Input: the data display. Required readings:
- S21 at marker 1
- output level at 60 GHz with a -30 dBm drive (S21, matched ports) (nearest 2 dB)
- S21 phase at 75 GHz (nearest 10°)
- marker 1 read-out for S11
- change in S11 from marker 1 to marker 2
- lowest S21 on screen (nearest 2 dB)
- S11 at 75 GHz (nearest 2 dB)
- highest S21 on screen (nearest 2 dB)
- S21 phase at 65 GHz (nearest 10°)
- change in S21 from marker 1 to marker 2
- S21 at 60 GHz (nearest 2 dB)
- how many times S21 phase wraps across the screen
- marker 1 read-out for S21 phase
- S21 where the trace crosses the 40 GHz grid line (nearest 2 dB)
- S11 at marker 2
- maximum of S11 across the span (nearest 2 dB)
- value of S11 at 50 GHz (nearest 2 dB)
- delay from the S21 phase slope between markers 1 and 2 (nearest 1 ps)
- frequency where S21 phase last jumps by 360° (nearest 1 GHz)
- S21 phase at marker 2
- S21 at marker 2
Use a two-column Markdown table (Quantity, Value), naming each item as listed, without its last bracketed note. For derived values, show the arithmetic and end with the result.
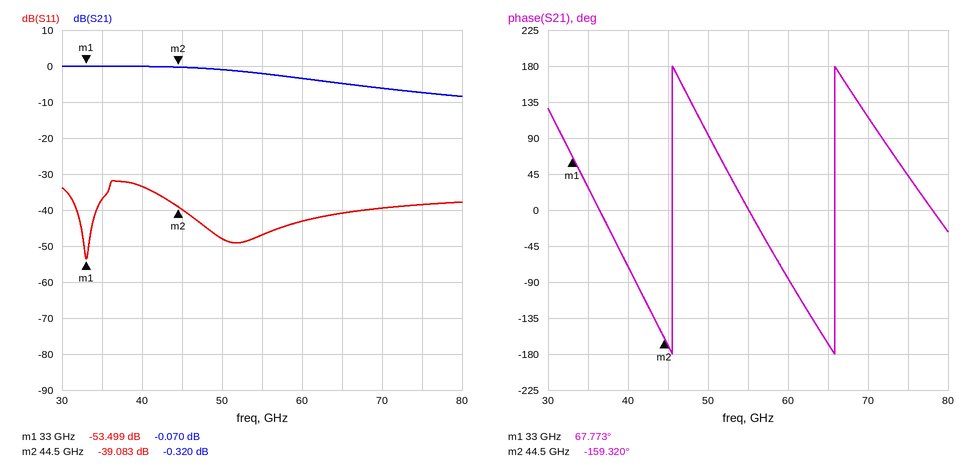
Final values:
| Quantity | Value |
|---|---|
| S21 at marker 1 | -0.070 dB |
| output level at 60 GHz with a -30 dBm drive (S21, matched ports) | -30 dBm + (-4 dB) = -34 dBm |
| S21 phase at 75 GHz | 40° |
| marker 1 read-out for S11 | -53.499 dB |
| change in S11 from marker 1 to marker 2 | -39.083 − (-53.499) = 14.416 dB |
| lowest S21 on screen | -8 dB |
| S11 at 75 GHz | -38 dB |
| highest S21 on screen | 0 dB |
| S21 phase at 65 GHz | -170° |
| change in S21 from marker 1 to marker 2 | -0.32 − (-0.07) = -0.250 dB |
| S21 at 60 GHz | -4 dB |
| how many times S21 phase wraps across the screen | 2 |
| marker 1 read-out for S21 phase | 67.773° |
| S21 where the trace crosses the 40 GHz grid line | 0 dB |
| S11 at marker 2 | -39.083 dB |
| maximum of S11 across the span | -32 dB |
| value of S11 at 50 GHz | -48 dB |
| delay from the S21 phase slope between markers 1 and 2 | −(-159.32° − (67.773°))/(360° × 11.5 GHz) ≈ 55 ps |
| frequency where S21 phase last jumps by 360° | 66 GHz |
| S21 phase at marker 2 | -159.320° |
| S21 at marker 2 | -0.320 dB |
